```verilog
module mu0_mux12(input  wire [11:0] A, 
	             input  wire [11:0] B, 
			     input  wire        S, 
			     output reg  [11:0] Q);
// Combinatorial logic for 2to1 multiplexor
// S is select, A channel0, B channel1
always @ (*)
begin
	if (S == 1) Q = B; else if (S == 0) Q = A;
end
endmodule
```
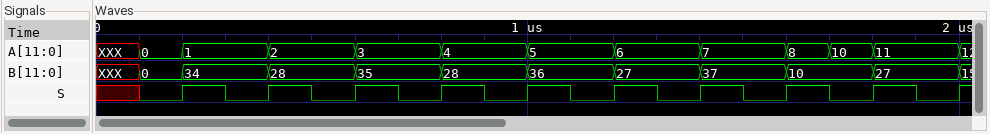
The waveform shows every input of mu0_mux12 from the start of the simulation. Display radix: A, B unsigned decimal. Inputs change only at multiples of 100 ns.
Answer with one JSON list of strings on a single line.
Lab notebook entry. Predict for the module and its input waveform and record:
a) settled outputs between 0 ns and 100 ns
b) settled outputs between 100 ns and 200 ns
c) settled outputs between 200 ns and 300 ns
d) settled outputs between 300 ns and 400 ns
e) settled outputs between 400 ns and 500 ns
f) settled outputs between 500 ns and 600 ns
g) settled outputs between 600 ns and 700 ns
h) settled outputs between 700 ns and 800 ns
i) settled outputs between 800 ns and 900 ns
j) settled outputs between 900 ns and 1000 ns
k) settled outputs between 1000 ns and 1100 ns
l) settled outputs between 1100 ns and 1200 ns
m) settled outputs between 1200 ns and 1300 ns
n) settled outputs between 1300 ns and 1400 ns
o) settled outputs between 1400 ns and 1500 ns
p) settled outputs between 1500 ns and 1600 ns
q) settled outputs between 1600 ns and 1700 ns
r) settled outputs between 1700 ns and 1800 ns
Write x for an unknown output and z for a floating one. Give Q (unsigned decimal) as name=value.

["Q=x", "Q=0", "Q=34", "Q=1", "Q=28", "Q=2", "Q=35", "Q=3", "Q=28", "Q=4", "Q=36", "Q=5", "Q=27", "Q=6", "Q=37", "Q=7", "Q=10", "Q=10"]
